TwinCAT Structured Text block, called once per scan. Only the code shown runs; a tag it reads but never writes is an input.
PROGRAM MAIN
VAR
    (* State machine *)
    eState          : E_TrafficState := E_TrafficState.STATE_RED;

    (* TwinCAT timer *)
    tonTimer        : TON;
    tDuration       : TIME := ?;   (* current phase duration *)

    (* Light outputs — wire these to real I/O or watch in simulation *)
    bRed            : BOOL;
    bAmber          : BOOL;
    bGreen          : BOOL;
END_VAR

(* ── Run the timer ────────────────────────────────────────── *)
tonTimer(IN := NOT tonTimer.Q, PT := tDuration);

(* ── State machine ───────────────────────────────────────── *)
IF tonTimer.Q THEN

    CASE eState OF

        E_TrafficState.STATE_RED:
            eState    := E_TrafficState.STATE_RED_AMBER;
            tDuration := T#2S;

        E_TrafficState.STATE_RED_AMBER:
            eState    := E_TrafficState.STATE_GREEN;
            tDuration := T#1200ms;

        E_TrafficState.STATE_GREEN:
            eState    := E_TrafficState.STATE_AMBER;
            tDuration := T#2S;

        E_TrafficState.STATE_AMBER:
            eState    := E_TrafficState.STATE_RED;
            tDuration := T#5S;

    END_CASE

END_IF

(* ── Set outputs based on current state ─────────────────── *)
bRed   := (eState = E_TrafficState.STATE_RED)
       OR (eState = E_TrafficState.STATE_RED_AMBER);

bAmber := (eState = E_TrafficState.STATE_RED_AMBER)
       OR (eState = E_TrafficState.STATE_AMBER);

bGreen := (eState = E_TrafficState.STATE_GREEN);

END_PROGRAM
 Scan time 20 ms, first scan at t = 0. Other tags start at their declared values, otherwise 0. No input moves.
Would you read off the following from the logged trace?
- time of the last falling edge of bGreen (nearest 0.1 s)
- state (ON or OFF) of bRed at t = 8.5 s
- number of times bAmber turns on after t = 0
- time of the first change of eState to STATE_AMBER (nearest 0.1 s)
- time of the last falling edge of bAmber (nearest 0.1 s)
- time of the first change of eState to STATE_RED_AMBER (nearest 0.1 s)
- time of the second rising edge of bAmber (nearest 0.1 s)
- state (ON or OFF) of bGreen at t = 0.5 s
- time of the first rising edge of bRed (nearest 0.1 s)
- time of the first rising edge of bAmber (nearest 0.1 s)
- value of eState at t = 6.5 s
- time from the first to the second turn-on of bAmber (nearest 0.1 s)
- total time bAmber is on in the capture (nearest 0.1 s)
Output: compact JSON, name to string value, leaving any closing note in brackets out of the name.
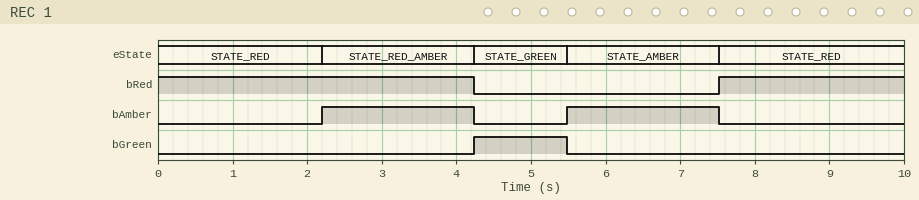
{"time of the last falling edge of bGreen": "5.5 s", "state (ON or OFF) of bRed at t = 8.5 s": "ON", "number of times bAmber turns on after t = 0": "2", "time of the first change of eState to STATE_AMBER": "5.5 s", "time of the last falling edge of bAmber": "7.5 s", "time of the first change of eState to STATE_RED_AMBER": "2.2 s", "time of the second rising edge of bAmber": "5.5 s", "state (ON or OFF) of bGreen at t = 0.5 s": "OFF", "time of the first rising edge of bRed": "7.5 s", "time of the first rising edge of bAmber": "2.2 s", "value of eState at t = 6.5 s": "STATE_AMBER", "time from the first to the second turn-on of bAmber": "3.3 s", "total time bAmber is on in the capture": "4.1 s"}
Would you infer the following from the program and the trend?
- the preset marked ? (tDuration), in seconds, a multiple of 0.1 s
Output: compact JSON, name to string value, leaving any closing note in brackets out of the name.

{"the preset marked ? (tDuration), in seconds, a multiple of 0.1 s": "2.2 s"}
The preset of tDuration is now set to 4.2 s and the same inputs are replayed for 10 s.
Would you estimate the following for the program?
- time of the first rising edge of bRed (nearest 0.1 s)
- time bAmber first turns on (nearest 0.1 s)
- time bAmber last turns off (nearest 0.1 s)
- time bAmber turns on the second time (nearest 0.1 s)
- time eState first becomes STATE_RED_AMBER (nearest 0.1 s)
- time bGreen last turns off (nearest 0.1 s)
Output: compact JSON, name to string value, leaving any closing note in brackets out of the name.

{"time of the first rising edge of bRed": "9.5 s", "time bAmber first turns on": "4.2 s", "time bAmber last turns off": "9.5 s", "time bAmber turns on the second time": "7.5 s", "time eState first becomes STATE_RED_AMBER": "4.2 s", "time bGreen last turns off": "7.5 s"}
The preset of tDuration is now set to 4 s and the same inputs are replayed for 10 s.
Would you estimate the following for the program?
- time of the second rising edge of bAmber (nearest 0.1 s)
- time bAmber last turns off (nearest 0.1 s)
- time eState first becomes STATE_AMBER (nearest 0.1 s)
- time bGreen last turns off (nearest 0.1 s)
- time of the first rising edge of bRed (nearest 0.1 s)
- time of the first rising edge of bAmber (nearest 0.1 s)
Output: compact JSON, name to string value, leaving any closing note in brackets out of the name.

{"time of the second rising edge of bAmber": "7.3 s", "time bAmber last turns off": "9.3 s", "time eState first becomes STATE_AMBER": "7.3 s", "time bGreen last turns off": "7.3 s", "time of the first rising edge of bRed": "9.3 s", "time of the first rising edge of bAmber": "4.0 s"}
